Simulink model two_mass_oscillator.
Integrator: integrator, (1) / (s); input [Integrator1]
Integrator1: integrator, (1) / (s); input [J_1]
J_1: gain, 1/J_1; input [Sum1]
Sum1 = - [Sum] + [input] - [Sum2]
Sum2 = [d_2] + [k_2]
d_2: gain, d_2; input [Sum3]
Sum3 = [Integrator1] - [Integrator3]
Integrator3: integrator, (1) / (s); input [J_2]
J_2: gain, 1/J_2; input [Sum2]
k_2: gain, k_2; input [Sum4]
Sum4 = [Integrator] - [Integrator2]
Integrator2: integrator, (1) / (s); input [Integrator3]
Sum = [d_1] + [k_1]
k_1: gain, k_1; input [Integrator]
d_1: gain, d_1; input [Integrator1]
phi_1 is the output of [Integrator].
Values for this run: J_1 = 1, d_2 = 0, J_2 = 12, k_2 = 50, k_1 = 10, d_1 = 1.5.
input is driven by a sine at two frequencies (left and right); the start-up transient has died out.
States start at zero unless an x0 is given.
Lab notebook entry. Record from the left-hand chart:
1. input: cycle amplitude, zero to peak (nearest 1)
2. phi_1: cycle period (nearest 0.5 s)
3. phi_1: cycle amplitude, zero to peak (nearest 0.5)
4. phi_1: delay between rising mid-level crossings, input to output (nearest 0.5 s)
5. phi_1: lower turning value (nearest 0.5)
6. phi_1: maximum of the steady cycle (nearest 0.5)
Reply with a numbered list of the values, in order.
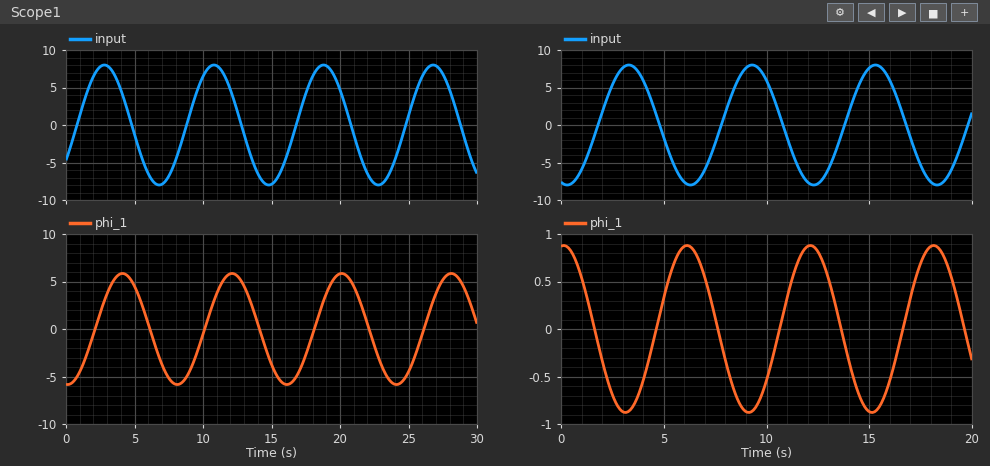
1. 8
2. 8.0 s
3. 6.0
4. 1.5 s
5. -6.0
6. 6.0
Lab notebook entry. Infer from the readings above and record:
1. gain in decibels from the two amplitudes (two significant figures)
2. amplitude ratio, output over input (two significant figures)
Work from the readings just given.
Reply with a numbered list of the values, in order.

1. -2.5 dB
2. 0.75
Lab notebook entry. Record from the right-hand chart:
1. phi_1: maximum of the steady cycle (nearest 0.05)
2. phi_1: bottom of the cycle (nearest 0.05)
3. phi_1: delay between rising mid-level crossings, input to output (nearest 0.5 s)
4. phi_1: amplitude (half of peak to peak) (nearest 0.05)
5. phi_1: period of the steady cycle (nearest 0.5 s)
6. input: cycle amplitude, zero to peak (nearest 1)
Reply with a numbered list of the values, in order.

1. 0.90
2. -0.90
3. 3.0 s
4. 0.90
5. 6.0 s
6. 8
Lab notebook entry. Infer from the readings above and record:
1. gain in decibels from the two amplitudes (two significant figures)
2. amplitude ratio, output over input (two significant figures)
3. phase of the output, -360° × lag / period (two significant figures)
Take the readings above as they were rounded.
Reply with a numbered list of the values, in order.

1. -19 dB
2. 0.11
3. -180°
